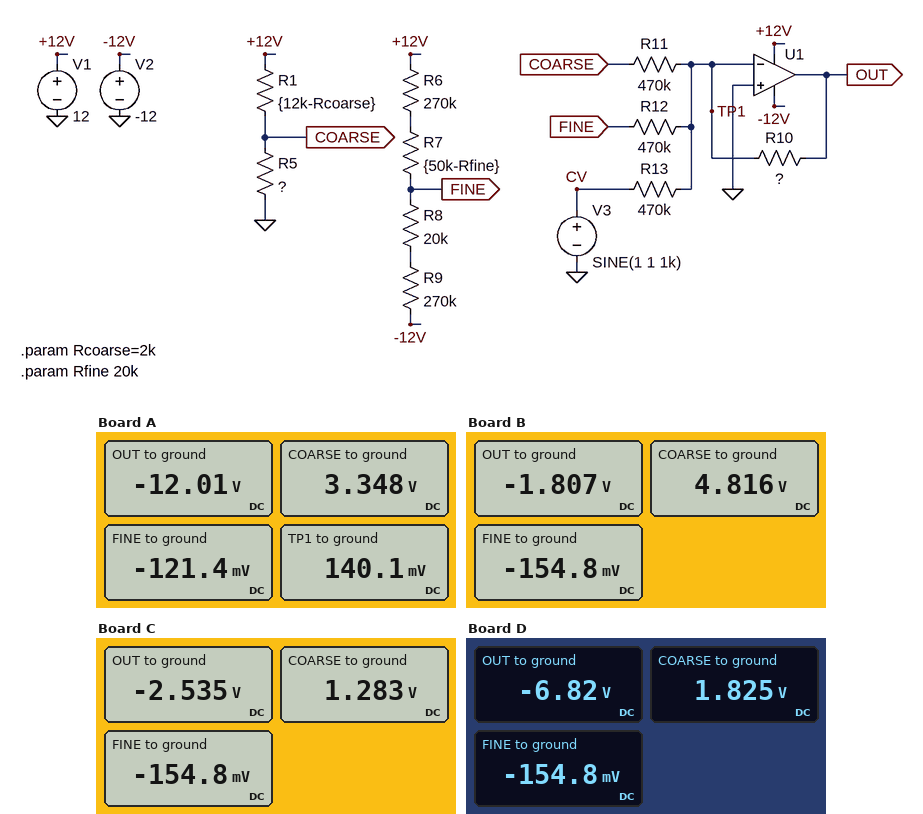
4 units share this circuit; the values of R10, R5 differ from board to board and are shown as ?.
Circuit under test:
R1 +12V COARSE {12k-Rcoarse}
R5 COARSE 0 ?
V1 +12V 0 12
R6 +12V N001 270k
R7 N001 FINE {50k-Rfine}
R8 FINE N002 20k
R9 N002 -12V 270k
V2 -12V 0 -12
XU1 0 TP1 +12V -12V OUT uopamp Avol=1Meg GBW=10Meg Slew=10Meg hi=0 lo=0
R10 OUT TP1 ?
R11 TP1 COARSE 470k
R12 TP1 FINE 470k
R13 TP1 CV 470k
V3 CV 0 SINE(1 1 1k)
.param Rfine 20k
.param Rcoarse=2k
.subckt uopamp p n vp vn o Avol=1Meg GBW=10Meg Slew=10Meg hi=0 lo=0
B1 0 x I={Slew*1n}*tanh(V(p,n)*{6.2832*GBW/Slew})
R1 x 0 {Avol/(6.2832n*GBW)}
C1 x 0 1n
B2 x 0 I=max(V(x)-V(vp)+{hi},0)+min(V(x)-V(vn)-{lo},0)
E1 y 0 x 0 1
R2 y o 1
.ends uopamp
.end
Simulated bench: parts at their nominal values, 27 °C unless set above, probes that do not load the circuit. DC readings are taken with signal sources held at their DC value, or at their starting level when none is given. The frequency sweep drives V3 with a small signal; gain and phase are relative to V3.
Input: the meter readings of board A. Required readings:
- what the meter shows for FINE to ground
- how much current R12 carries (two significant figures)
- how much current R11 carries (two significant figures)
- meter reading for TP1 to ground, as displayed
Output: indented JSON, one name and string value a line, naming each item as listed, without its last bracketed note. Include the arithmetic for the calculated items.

{
  "what the meter shows for FINE to ground": "-121.4 mV",
  "how much current R12 carries": "(140.1 mV - (-121.4 mV)) / 470 kΩ = 560 nA",
  "how much current R11 carries": "(3.348 V - 140.1 mV) / 470 kΩ = 6.8 µA",
  "meter reading for TP1 to ground, as displayed": "140.1 mV"
}
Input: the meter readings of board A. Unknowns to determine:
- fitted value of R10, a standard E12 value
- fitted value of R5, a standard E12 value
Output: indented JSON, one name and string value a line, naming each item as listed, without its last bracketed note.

{
  "fitted value of R10, a standard E12 value": "1.5 MΩ",
  "fitted value of R5, a standard E12 value": "3.9 kΩ"
}
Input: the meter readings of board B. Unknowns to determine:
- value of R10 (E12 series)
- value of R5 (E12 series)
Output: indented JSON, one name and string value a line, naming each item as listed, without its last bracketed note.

{
  "value of R10": "150 kΩ",
  "value of R5": "6.8 kΩ"
}
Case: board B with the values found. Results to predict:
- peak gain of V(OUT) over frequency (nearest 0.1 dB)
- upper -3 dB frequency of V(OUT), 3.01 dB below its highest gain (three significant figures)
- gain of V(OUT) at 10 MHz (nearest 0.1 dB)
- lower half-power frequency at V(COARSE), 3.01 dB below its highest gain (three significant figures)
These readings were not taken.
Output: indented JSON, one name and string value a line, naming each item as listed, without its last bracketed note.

{
  "peak gain of V(OUT) over frequency": "-9.9 dB",
  "upper -3 dB frequency of V(OUT), 3.01 dB below its highest gain": "5.32 MHz",
  "gain of V(OUT) at 10 MHz": "-16.5 dB",
  "lower half-power frequency at V(COARSE), 3.01 dB below its highest gain": "5.32 MHz"
}
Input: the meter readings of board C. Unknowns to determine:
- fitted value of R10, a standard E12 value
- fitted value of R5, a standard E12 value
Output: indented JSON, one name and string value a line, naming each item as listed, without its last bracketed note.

{
  "fitted value of R10, a standard E12 value": "560 kΩ",
  "fitted value of R5, a standard E12 value": "1.2 kΩ"
}
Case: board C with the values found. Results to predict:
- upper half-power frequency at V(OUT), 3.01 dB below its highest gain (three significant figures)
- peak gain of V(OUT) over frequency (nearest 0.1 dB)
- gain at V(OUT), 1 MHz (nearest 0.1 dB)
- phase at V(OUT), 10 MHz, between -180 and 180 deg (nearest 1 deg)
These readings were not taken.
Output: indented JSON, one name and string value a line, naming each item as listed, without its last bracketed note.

{
  "upper half-power frequency at V(OUT), 3.01 dB below its highest gain": "2.33 MHz",
  "peak gain of V(OUT) over frequency": "1.5 dB",
  "gain at V(OUT), 1 MHz": "0.8 dB",
  "phase at V(OUT), 10 MHz, between -180 and 180 deg": "103 deg"
}
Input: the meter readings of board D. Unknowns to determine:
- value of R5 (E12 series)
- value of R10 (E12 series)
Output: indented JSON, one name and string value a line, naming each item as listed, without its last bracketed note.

{
  "value of R5": "1.8 kΩ",
  "value of R10": "1.2 MΩ"
}
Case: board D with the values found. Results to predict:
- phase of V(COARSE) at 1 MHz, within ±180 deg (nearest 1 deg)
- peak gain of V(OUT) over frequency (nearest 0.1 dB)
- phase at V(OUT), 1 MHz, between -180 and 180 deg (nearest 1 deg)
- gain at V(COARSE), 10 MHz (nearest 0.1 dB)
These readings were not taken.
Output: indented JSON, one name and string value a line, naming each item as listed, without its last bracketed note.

{
  "phase of V(COARSE) at 1 MHz, within ±180 deg": "51 deg",
  "peak gain of V(OUT) over frequency": "8.1 dB",
  "phase at V(OUT), 1 MHz, between -180 and 180 deg": "141 deg",
  "gain at V(COARSE), 10 MHz": "-59.8 dB"
}
